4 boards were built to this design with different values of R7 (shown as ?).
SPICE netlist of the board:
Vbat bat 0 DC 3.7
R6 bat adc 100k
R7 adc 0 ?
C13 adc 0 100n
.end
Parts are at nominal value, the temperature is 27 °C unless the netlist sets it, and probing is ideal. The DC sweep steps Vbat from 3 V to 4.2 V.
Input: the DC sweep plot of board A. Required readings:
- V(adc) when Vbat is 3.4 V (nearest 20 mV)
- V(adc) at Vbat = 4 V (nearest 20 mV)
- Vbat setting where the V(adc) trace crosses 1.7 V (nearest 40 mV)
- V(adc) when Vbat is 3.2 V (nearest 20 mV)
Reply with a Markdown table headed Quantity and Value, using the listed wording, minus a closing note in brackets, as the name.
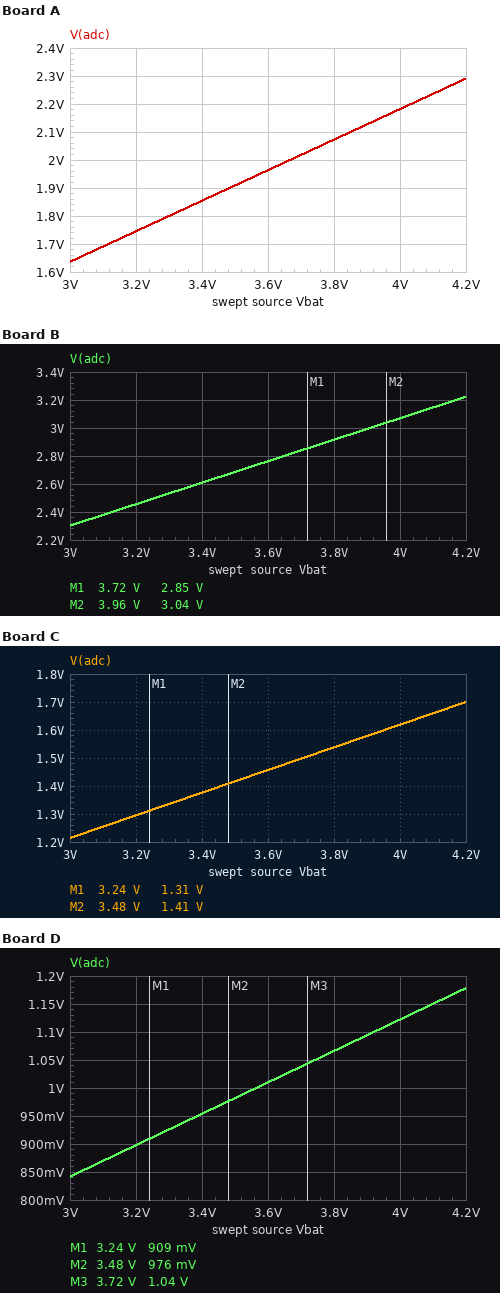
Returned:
| Quantity | Value |
|---|---|
| V(adc) when Vbat is 3.4 V | 1.86 V |
| V(adc) at Vbat = 4 V | 2.18 V |
| Vbat setting where the V(adc) trace crosses 1.7 V | 3.12 V |
| V(adc) when Vbat is 3.2 V | 1.74 V |
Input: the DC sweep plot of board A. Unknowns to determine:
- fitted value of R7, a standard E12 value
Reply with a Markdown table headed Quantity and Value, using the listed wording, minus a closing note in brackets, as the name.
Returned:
| Quantity | Value |
|---|---|
| fitted value of R7, a standard E12 value | 120 kΩ |
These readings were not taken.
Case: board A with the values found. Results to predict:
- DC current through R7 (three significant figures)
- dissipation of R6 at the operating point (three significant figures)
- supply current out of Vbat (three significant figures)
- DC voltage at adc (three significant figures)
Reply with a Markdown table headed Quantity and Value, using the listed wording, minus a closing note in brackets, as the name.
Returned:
| Quantity | Value |
|---|---|
| DC current through R7 | 16.8 µA |
| dissipation of R6 at the operating point | 28.3 µW |
| supply current out of Vbat | 16.8 µA |
| DC voltage at adc | 2.02 V |
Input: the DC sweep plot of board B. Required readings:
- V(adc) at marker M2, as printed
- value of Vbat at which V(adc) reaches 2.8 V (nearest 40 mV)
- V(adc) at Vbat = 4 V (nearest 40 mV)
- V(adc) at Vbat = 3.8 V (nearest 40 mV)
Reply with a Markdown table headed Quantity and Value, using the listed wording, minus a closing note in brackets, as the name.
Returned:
| Quantity | Value |
|---|---|
| V(adc) at marker M2, as printed | 3.04 V |
| value of Vbat at which V(adc) reaches 2.8 V | 3.64 V |
| V(adc) at Vbat = 4 V | 3.08 V |
| V(adc) at Vbat = 3.8 V | 2.92 V |
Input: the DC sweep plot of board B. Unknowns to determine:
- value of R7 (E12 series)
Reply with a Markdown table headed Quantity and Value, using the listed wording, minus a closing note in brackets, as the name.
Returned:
| Quantity | Value |
|---|---|
| value of R7 | 330 kΩ |
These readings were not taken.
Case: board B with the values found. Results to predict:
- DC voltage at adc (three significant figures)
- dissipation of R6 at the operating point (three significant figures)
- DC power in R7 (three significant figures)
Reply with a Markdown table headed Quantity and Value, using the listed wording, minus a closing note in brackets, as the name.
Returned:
| Quantity | Value |
|---|---|
| DC voltage at adc | 2.84 V |
| dissipation of R6 at the operating point | 7.40 µW |
| DC power in R7 | 24.4 µW |
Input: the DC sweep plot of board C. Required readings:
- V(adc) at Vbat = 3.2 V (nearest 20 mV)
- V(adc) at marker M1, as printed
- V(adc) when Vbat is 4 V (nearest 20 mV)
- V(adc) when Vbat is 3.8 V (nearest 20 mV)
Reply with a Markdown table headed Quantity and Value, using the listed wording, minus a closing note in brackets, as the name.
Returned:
| Quantity | Value |
|---|---|
| V(adc) at Vbat = 3.2 V | 1.30 V |
| V(adc) at marker M1, as printed | 1.31 V |
| V(adc) when Vbat is 4 V | 1.62 V |
| V(adc) when Vbat is 3.8 V | 1.54 V |
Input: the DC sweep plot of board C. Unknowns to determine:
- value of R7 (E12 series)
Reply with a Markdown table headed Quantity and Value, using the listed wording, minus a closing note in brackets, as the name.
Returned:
| Quantity | Value |
|---|---|
| value of R7 | 68 kΩ |
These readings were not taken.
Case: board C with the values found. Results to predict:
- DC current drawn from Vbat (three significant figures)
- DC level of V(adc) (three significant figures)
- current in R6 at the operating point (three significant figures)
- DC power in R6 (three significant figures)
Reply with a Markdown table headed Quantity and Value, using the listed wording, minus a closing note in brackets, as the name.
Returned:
| Quantity | Value |
|---|---|
| DC current drawn from Vbat | 22.0 µA |
| DC level of V(adc) | 1.50 V |
| current in R6 at the operating point | 22.0 µA |
| DC power in R6 | 48.5 µW |
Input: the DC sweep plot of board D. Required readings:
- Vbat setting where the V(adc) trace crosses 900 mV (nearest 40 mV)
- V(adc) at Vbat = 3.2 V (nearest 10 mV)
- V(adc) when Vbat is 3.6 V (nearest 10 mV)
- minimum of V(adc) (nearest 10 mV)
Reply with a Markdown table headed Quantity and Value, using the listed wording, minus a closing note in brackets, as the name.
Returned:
| Quantity | Value |
|---|---|
| Vbat setting where the V(adc) trace crosses 900 mV | 3.20 V |
| V(adc) at Vbat = 3.2 V | 900 mV |
| V(adc) when Vbat is 3.6 V | 1.01 V |
| minimum of V(adc) | 840 mV |
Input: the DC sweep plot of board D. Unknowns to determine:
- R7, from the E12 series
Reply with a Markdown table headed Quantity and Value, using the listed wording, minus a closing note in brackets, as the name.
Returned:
| Quantity | Value |
|---|---|
| R7, from the E12 series | 39 kΩ |
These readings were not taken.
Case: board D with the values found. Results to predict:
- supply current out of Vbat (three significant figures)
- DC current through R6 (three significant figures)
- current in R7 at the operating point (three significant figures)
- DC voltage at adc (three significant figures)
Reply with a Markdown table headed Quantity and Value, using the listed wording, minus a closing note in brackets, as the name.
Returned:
| Quantity | Value |
|---|---|
| supply current out of Vbat | 26.6 µA |
| DC current through R6 | 26.6 µA |
| current in R7 at the operating point | 26.6 µA |
| DC voltage at adc | 1.04 V |
